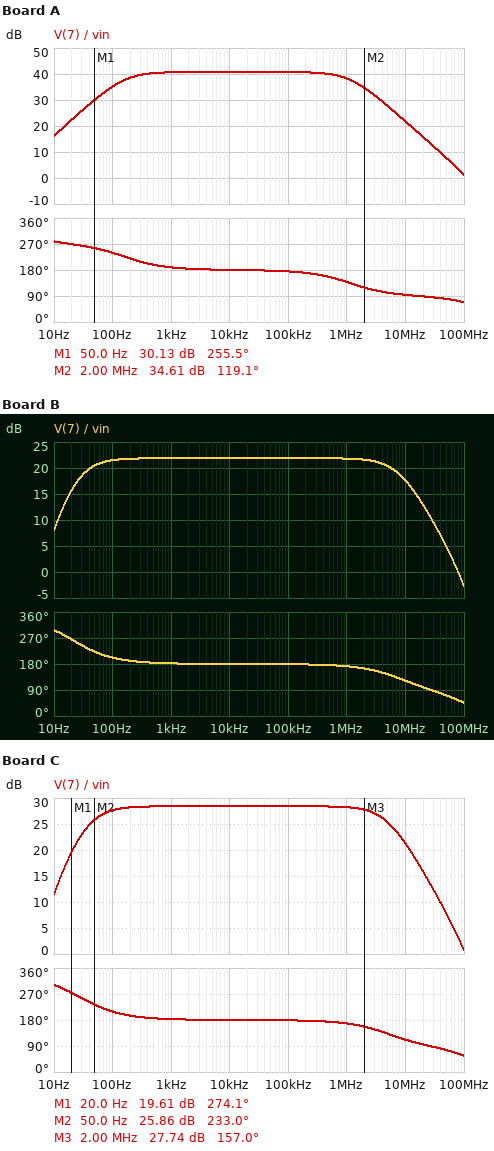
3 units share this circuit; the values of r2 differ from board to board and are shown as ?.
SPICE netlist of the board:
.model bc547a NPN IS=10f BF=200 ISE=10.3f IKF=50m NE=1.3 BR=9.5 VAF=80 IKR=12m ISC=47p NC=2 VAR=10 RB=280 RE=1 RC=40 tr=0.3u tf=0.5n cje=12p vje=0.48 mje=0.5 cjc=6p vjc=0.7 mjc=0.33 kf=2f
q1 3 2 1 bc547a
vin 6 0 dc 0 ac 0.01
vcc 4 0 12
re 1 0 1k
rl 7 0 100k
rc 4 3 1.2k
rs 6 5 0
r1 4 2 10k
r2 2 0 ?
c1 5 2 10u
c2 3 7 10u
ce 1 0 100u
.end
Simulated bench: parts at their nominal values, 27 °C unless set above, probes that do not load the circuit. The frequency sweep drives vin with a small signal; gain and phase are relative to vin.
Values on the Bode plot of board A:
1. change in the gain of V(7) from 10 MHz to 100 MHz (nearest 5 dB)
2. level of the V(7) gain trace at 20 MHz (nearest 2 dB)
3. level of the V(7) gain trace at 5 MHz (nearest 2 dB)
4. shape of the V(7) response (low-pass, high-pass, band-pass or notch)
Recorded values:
-20 dB
16 dB
28 dB
band-pass
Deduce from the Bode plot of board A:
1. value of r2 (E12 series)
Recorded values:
6.8 kΩ
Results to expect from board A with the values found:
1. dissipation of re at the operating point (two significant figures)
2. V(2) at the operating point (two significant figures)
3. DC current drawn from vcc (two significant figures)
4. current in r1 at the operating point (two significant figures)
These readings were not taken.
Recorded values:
16 mW
4.7 V
4.7 mA
730 µA
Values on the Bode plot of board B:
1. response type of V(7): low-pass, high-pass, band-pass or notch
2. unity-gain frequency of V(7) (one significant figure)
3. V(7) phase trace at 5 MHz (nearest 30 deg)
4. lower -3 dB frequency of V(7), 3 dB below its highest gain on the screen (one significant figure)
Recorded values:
band-pass
80 MHz
150 deg
30 Hz
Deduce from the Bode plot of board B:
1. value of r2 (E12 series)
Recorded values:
820 Ω
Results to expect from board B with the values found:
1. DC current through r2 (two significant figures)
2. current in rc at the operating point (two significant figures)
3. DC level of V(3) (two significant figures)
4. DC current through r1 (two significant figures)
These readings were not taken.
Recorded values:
1.1 mA
280 µA
12 V
1.1 mA
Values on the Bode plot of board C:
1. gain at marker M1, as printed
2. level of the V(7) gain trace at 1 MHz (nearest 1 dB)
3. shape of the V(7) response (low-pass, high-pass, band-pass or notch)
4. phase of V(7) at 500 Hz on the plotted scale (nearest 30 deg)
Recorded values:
19.61 dB
28 dB
band-pass
180 deg
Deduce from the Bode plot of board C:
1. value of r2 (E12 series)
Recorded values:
1.2 kΩ
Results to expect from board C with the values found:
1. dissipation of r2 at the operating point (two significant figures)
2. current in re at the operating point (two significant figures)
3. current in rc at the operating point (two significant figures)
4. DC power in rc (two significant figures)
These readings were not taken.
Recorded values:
1.4 mW
640 µA
630 µA
480 µW
